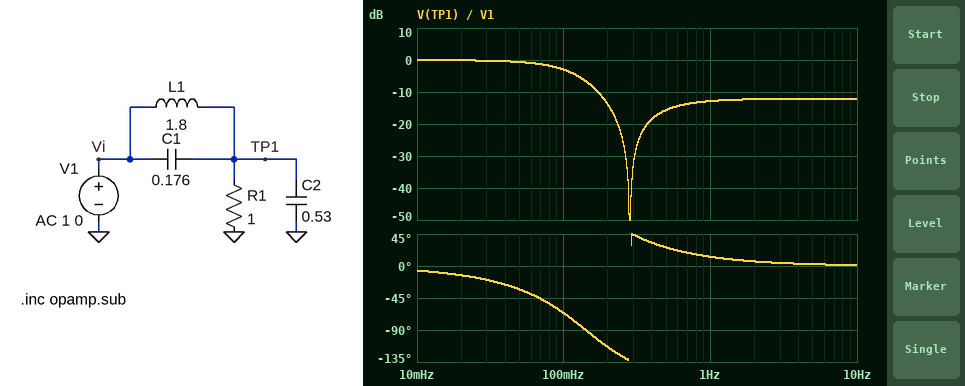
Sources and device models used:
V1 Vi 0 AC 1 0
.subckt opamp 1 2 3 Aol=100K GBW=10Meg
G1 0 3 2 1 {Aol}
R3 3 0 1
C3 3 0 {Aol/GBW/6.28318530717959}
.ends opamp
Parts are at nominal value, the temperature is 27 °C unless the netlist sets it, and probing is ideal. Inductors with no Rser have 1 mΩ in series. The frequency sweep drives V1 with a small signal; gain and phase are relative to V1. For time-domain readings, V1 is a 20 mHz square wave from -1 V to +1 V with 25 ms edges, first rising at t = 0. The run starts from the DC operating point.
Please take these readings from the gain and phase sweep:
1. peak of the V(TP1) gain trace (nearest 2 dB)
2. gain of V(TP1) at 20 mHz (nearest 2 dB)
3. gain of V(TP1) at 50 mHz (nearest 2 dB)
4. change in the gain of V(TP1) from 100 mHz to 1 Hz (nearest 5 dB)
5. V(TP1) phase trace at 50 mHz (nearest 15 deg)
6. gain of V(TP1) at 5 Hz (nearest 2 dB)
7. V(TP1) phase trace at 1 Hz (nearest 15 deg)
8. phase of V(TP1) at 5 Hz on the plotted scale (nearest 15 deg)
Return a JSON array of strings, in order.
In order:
["0 dB", "0 dB", "0 dB", "-10 dB", "-30 deg", "-12 dB", "15 deg", "0 deg"]
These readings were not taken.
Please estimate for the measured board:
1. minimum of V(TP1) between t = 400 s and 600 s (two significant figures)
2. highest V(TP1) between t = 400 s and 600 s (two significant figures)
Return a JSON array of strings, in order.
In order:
["-1.0 V", "1.0 V"]
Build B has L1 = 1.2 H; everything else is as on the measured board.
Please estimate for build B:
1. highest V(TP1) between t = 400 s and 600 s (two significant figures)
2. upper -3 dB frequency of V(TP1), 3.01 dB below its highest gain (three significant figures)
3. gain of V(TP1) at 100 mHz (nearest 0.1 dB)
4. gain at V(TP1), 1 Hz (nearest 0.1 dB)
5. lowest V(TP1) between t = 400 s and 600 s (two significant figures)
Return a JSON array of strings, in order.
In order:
["1.1 V", "149 mHz", "-0.8 dB", "-13.1 dB", "-1.1 V"]
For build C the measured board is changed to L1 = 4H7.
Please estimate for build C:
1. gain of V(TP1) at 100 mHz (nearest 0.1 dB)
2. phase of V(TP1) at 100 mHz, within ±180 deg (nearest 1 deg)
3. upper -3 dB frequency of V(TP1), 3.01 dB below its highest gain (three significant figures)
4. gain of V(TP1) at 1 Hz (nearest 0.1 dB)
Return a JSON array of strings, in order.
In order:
["-12.9 dB", "-96 deg", "36.3 mHz", "-12.5 dB"]
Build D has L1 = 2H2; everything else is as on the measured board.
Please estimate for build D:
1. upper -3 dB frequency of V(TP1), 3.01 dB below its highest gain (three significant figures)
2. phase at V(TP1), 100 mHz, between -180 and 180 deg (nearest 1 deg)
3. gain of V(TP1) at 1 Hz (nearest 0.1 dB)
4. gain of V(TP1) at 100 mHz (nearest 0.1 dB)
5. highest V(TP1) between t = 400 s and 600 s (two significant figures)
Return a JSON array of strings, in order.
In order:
["81.3 mHz", "-74 deg", "-12.7 dB", "-4.6 dB", "1.0 V"]
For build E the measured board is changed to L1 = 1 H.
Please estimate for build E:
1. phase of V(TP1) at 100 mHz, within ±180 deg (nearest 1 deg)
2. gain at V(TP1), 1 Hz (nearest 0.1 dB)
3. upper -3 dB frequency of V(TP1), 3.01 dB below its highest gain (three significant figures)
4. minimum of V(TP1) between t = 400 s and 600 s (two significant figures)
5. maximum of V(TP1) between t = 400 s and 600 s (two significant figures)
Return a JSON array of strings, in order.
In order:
["-41 deg", "-13.3 dB", "175 mHz", "-1.2 V", "1.2 V"]
